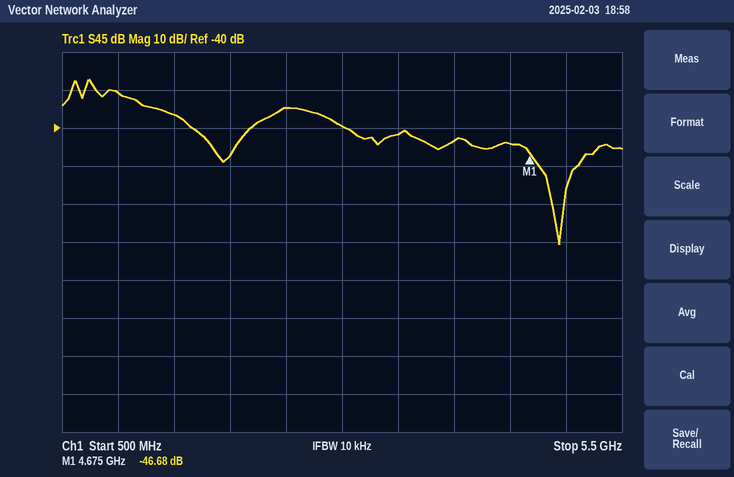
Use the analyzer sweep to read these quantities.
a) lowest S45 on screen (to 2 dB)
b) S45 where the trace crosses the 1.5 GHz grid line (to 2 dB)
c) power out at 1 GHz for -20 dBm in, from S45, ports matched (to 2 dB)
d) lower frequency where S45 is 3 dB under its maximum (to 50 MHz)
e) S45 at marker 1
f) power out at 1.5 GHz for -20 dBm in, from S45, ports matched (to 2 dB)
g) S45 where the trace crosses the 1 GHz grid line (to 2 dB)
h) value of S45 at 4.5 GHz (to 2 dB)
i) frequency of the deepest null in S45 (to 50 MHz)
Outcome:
-70 dB
-36 dB
-50 dBm
700 MHz
-46.68 dB
-56 dBm
-30 dB
-44 dB
4.95 GHz
